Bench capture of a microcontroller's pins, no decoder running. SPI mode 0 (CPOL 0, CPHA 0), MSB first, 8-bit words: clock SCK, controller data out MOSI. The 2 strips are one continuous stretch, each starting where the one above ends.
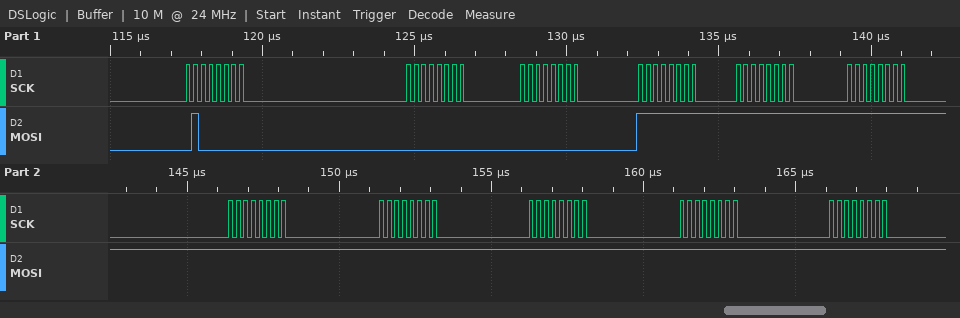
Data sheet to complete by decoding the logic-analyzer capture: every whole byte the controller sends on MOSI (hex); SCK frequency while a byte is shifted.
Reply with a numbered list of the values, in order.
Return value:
1. 0x40 0x00 0x00 0xFF 0xFF 0xFF 0xFF 0xFF 0xFF 0xFF 0xFF
2. 4 MHz
